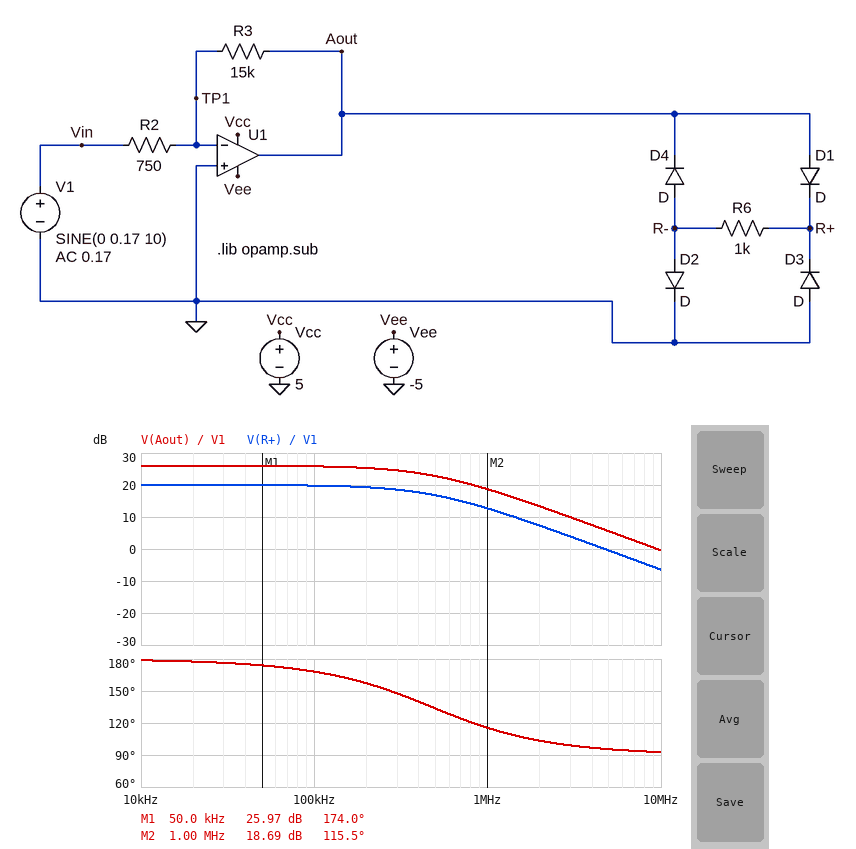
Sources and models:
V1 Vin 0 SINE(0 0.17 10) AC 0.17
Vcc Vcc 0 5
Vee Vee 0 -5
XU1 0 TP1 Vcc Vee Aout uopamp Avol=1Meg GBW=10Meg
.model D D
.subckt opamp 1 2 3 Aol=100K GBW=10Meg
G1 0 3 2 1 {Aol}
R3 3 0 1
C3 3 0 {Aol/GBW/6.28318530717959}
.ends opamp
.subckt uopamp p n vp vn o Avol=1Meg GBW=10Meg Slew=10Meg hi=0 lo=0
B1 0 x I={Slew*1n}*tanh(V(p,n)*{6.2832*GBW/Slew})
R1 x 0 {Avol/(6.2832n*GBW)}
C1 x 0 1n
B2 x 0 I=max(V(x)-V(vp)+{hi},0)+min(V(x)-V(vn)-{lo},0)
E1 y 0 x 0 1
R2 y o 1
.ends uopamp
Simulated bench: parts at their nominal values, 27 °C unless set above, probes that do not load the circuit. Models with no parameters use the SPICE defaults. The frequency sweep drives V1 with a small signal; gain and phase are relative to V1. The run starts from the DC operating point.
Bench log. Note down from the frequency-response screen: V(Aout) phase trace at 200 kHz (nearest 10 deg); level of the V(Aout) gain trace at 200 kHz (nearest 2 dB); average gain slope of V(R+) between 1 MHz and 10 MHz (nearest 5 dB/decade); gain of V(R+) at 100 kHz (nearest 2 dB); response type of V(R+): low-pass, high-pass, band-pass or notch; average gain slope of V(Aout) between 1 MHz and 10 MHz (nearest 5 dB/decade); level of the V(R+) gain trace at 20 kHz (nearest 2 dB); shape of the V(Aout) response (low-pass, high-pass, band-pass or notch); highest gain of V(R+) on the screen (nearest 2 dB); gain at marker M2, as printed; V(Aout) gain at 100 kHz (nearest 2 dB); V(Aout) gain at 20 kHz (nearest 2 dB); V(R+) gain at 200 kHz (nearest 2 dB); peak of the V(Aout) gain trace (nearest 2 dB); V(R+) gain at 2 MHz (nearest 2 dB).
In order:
160 deg
26 dB
-20 dB/decade
20 dB
low-pass
-20 dB/decade
20 dB
low-pass
20 dB
18.69 dB
26 dB
26 dB
20 dB
26 dB
8 dB
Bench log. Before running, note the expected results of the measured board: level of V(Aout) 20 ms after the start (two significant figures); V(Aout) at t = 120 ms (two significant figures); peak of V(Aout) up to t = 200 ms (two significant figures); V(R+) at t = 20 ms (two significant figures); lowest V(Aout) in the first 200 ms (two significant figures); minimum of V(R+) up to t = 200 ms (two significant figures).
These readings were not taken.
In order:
-3.2 V
-3.2 V
3.4 V
-670 mV
-3.4 V
-670 mV
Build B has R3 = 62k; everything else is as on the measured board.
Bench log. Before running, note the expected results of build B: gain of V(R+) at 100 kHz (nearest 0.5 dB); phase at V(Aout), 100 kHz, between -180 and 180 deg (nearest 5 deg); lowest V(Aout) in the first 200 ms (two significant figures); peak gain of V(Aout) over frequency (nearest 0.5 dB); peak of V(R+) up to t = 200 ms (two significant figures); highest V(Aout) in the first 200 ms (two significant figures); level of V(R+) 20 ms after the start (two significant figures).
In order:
30.0 dB
140 deg
-5.0 V
38.5 dB
4.3 V
5.0 V
-690 mV
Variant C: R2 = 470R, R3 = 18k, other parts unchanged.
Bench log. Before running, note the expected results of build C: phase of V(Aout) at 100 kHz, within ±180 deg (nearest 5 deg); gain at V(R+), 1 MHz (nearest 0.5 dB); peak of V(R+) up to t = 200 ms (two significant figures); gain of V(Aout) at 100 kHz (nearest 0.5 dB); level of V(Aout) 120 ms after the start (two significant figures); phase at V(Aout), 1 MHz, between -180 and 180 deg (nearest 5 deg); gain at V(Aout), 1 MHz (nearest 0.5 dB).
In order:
160 deg
13.5 dB
4.3 V
31.0 dB
-5.0 V
105 deg
19.5 dB
